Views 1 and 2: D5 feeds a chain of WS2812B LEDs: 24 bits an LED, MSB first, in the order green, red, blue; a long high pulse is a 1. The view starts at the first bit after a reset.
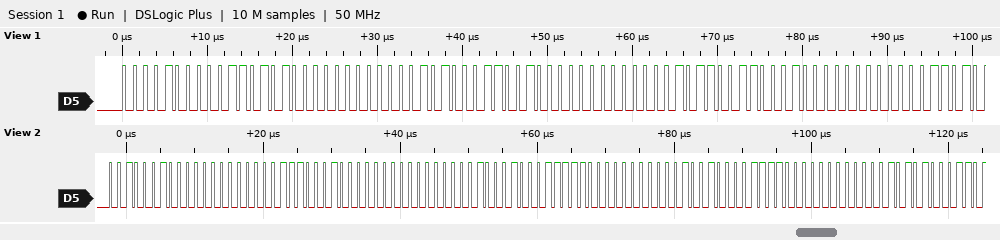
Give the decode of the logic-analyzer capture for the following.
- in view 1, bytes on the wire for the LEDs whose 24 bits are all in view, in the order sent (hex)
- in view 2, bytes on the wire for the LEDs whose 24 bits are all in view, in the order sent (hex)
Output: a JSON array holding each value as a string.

["08 35 00 0A 32 00 0B 31 00", "22 00 0E 20 00 11 1F 00 12 1E 00 15"]
